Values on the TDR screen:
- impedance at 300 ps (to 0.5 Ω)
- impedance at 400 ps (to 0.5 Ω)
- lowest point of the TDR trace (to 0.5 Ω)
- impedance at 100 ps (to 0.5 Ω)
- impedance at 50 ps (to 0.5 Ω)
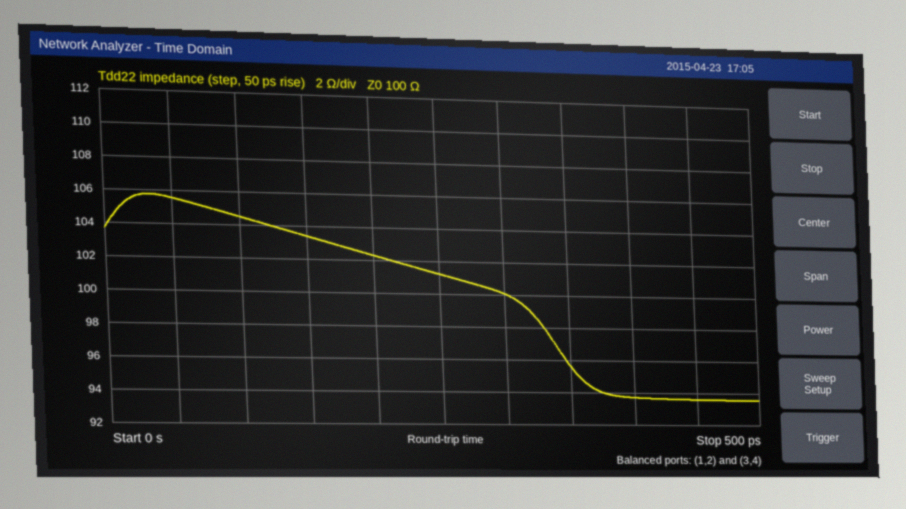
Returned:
100.0 Ω
93.5 Ω
93.5 Ω
104.5 Ω
105.5 Ω
